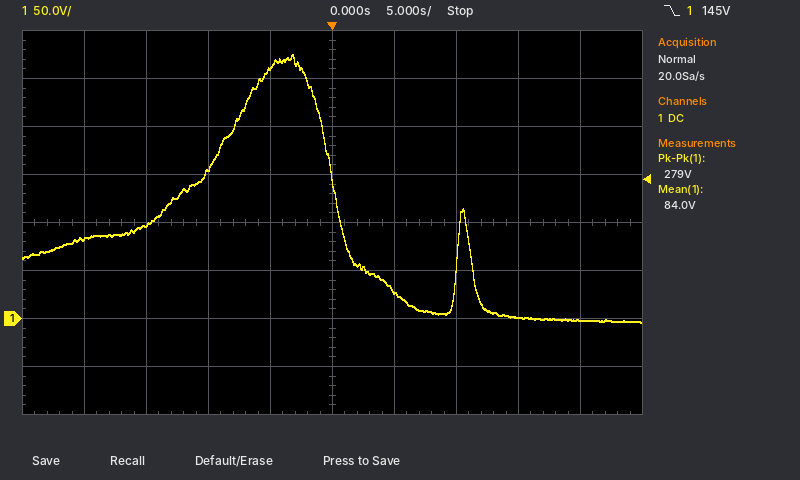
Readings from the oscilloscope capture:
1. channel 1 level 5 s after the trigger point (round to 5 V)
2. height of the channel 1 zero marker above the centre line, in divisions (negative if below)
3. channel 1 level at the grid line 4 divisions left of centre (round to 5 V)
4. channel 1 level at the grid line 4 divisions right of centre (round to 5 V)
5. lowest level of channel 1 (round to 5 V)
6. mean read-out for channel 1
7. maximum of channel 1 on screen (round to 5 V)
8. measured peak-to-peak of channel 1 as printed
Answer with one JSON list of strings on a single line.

["30 V", "-2.0 div", "85 V", "0 V", "-5 V", "84.0 V", "275 V", "279 V"]
